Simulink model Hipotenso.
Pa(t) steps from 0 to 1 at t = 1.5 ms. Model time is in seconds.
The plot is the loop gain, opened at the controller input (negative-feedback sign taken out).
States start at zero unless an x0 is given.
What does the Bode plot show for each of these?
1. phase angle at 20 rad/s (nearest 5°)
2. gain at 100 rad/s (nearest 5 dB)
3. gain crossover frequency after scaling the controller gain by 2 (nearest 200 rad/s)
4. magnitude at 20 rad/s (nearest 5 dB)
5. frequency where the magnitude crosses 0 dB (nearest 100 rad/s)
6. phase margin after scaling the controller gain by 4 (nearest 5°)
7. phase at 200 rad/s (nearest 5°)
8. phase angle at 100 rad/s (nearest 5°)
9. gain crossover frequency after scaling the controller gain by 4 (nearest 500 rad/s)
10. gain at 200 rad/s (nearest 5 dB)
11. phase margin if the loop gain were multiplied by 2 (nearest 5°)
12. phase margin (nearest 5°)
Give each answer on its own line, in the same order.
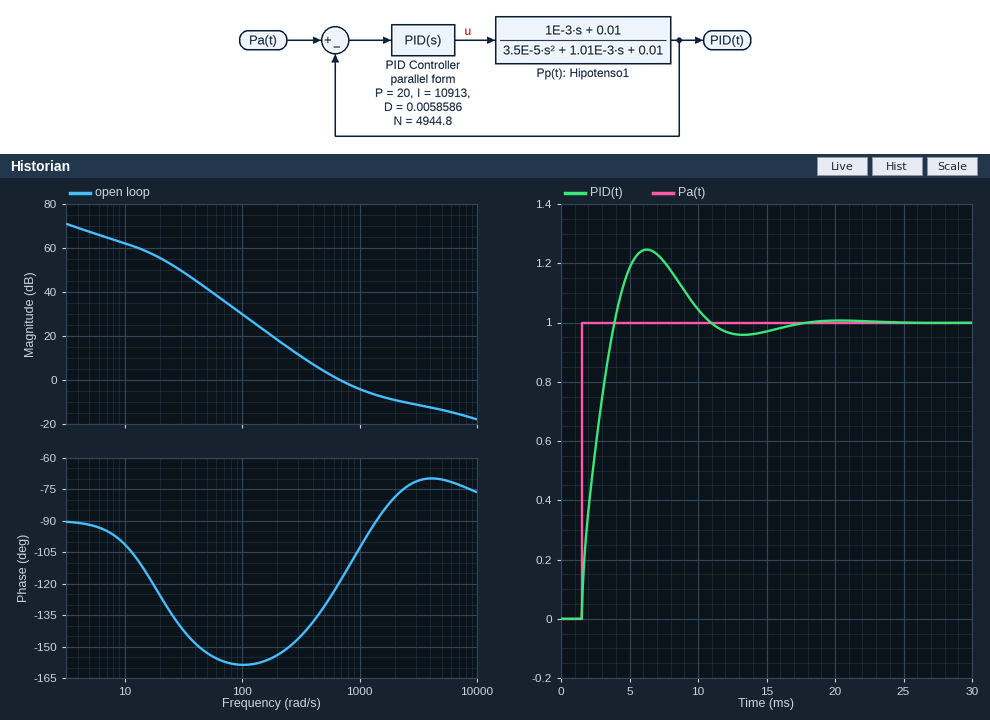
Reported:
-125°
30 dB
1200 rad/s
55 dB
700 rad/s
110°
-155°
-160°
3500 rad/s
20 dB
85°
60°
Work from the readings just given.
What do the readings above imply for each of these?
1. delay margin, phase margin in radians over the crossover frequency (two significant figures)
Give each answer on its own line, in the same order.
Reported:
0.0015 s
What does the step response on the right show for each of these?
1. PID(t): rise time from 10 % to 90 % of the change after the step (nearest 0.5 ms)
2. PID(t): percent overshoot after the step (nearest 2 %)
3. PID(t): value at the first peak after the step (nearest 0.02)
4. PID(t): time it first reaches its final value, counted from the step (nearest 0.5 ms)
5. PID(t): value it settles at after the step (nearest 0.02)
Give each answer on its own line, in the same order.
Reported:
2.0 ms
24 %
1.24
2.5 ms
1.00
